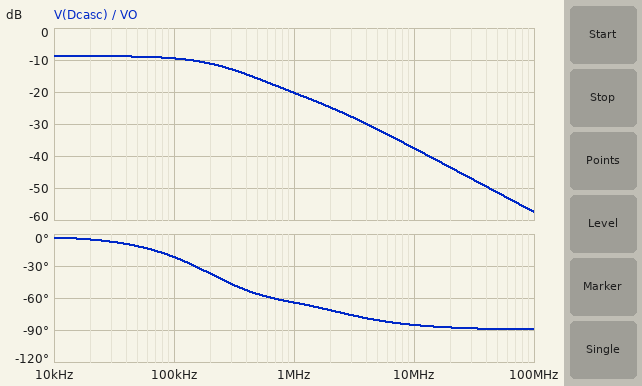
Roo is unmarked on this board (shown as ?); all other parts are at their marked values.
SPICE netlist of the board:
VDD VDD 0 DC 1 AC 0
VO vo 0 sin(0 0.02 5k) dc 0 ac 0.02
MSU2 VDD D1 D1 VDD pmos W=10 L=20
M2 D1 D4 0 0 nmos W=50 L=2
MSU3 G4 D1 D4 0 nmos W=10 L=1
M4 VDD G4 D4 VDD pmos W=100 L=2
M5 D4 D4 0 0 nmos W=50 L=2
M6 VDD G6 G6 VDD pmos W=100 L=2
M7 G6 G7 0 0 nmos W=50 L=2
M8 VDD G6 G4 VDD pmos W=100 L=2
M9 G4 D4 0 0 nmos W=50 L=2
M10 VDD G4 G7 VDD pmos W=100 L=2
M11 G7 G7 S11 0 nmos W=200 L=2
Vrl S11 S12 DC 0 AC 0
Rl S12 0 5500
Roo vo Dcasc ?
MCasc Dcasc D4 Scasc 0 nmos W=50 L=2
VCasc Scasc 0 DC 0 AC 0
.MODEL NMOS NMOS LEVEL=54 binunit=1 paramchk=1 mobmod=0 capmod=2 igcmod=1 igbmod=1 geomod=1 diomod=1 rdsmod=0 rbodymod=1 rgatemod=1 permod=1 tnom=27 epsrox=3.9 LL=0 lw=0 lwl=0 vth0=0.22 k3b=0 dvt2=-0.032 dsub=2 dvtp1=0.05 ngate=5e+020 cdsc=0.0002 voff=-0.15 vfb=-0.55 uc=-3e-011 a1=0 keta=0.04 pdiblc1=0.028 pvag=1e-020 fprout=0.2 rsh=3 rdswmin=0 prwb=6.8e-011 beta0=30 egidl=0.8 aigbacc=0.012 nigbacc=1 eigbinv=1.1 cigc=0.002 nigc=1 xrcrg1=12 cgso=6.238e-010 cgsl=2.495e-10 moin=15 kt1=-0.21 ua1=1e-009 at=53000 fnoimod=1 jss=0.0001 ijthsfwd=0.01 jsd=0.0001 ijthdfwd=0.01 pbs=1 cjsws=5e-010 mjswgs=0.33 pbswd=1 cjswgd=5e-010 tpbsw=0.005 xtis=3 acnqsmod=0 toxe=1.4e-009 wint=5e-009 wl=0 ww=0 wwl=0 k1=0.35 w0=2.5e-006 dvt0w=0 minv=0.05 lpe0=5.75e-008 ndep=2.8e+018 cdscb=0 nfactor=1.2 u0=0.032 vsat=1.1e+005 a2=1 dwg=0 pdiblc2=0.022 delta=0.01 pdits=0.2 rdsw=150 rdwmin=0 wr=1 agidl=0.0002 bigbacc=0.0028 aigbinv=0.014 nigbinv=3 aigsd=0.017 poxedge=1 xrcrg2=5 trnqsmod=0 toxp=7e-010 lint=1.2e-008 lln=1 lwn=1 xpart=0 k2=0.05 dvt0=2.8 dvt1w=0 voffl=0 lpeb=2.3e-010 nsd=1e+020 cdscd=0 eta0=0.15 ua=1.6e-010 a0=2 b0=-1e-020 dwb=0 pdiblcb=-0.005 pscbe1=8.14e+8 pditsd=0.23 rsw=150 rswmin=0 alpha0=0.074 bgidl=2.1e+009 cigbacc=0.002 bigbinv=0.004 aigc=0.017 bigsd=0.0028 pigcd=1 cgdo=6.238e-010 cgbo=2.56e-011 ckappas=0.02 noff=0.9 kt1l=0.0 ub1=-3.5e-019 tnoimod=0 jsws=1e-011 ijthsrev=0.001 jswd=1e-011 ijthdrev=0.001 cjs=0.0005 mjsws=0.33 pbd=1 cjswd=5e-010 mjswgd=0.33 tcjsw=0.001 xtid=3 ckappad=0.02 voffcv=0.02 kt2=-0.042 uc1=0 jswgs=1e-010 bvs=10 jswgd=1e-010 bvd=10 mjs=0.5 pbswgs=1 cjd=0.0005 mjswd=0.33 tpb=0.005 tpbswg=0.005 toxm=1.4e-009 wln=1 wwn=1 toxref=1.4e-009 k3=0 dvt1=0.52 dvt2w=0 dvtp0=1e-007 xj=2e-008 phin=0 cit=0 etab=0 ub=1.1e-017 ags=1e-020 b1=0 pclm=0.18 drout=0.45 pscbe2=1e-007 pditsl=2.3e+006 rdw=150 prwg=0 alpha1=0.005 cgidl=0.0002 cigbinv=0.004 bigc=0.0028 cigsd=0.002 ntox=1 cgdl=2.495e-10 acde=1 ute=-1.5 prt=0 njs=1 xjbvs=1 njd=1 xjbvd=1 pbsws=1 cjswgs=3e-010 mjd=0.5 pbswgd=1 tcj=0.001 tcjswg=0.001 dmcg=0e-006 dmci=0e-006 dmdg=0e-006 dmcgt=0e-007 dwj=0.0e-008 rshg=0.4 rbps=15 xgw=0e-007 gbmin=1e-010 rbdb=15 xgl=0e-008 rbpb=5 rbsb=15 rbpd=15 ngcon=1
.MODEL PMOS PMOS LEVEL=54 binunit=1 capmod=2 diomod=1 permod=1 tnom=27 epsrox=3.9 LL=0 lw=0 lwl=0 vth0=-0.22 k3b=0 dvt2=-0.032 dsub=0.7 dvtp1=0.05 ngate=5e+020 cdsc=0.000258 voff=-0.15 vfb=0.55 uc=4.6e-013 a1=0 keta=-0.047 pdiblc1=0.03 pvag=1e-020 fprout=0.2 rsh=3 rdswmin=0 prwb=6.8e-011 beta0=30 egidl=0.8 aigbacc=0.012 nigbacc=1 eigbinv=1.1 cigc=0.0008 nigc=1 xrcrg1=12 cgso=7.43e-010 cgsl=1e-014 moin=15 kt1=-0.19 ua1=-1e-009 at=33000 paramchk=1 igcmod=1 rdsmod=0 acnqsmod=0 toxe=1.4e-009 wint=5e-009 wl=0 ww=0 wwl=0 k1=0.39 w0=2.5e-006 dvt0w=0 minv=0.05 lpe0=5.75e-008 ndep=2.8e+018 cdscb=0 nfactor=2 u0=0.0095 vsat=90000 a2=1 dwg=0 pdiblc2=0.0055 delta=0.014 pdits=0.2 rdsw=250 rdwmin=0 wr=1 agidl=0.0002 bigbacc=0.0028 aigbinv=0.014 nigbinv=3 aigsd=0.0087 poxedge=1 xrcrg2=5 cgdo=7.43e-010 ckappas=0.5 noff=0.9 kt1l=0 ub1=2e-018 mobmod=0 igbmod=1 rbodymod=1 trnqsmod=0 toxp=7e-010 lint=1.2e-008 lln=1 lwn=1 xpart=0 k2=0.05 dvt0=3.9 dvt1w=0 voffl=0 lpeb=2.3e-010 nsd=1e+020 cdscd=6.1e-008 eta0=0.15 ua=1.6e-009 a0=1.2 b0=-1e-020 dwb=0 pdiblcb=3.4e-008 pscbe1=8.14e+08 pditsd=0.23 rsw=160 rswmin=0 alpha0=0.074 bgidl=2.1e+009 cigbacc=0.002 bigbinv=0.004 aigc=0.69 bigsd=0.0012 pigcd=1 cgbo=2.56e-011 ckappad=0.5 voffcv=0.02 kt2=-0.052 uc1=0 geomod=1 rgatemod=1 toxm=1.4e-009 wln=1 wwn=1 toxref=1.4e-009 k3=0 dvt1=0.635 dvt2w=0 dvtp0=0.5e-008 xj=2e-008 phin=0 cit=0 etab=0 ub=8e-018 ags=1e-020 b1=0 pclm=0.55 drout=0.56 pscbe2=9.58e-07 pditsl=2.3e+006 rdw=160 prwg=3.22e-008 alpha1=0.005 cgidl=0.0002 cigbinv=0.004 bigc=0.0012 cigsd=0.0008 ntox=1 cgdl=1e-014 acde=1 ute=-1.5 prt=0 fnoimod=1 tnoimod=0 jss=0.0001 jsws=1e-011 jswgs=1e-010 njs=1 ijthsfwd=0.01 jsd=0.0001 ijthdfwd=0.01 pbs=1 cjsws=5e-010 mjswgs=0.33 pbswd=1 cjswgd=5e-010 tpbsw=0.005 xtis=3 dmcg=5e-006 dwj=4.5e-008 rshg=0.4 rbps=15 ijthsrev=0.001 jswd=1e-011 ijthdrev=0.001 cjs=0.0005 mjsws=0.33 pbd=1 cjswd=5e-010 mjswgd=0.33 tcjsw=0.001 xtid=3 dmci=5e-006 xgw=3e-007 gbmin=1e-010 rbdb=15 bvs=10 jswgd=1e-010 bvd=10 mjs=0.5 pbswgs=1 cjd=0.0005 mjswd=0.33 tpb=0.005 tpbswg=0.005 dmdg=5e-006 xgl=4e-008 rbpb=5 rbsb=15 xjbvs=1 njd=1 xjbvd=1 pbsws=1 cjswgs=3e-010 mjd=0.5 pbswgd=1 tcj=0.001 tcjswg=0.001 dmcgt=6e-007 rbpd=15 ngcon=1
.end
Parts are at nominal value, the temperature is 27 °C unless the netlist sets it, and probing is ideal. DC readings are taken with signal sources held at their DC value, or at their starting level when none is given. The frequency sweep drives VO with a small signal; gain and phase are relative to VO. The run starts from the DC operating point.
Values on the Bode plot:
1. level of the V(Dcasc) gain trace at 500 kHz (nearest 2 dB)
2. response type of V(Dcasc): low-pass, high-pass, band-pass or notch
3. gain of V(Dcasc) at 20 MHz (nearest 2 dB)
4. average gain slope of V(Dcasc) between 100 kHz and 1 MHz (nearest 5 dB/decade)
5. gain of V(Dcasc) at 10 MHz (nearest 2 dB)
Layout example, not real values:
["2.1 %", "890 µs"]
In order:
["-16 dB", "low-pass", "-44 dB", "-10 dB/decade", "-38 dB"]
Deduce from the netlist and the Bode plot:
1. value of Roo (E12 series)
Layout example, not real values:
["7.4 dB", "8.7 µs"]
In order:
["33 Ω"]
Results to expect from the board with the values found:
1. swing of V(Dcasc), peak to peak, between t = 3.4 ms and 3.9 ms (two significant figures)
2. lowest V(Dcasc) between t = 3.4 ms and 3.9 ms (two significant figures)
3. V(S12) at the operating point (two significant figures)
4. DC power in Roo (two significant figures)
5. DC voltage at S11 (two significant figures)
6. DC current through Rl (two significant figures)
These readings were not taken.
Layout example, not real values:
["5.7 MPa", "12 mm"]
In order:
["15 mV", "730 mV", "71 mV", "17 mW", "71 mV", "13 µA"]
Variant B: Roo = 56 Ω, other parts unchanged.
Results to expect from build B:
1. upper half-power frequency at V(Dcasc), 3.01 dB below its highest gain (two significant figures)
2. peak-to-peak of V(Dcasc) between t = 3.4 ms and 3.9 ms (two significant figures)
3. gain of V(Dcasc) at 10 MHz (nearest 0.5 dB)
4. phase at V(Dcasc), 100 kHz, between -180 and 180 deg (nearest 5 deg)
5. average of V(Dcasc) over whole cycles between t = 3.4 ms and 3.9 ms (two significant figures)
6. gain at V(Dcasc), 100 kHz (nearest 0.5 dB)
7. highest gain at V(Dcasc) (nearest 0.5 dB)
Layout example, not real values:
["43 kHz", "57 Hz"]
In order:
["250 kHz", "6.6 mV", "-41.0 dB", "-15 deg", "860 mV", "-16.0 dB", "-14.5 dB"]
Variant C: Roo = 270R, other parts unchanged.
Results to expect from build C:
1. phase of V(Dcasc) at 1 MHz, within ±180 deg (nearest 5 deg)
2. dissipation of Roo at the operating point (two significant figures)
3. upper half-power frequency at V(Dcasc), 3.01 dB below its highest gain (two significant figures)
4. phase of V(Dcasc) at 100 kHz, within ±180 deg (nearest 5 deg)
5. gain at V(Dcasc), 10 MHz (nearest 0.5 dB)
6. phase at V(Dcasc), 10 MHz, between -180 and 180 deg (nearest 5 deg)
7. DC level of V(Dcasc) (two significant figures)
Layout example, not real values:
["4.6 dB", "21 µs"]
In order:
["-50 deg", "3.5 mW", "330 kHz", "-10 deg", "-54.0 dB", "-80 deg", "970 mV"]
